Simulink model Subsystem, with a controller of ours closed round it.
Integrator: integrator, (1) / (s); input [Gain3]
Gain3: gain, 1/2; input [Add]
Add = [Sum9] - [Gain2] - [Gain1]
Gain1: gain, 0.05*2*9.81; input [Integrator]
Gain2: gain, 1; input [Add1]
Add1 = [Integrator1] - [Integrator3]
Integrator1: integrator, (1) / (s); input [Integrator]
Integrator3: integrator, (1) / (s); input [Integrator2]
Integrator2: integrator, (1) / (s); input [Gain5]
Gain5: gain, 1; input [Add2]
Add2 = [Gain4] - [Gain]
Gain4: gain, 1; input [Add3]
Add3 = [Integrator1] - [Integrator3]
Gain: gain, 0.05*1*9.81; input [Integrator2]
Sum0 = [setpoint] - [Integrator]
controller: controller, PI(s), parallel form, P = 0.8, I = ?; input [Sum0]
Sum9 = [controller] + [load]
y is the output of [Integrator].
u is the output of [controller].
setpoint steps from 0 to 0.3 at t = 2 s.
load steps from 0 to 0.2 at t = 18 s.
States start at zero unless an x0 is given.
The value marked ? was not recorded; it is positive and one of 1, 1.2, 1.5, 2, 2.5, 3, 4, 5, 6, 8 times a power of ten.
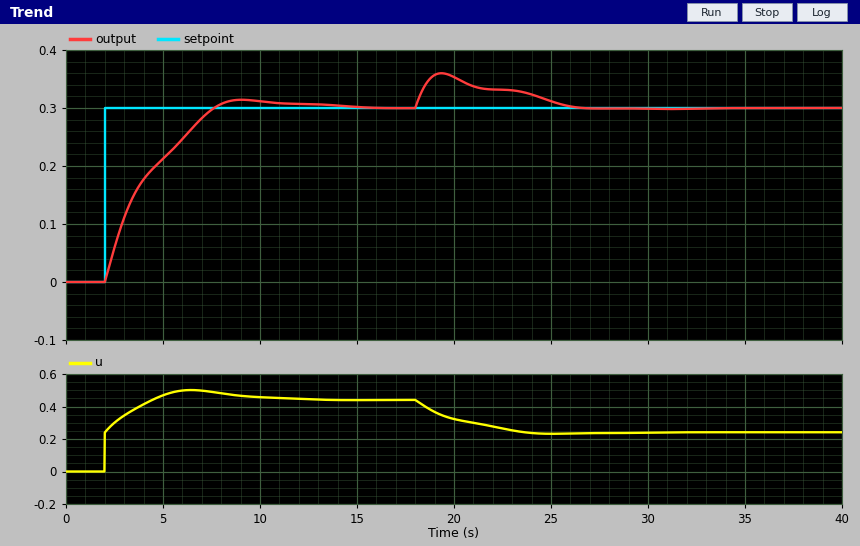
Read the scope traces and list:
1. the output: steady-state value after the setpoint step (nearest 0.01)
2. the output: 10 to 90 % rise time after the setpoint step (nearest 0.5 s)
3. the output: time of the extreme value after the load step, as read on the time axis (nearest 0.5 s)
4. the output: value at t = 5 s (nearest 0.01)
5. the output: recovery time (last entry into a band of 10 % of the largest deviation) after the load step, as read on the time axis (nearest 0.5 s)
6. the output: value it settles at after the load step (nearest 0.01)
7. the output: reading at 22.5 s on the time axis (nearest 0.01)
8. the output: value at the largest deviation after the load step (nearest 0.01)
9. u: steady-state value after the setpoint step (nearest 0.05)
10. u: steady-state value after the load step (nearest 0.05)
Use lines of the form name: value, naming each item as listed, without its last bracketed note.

the output: steady-state value after the setpoint step: 0.30
the output: 10 to 90 % rise time after the setpoint step: 4.5 s
the output: time of the extreme value after the load step, as read on the time axis: 19.5 s
the output: value at t = 5 s: 0.21
the output: recovery time (last entry into a band of 10 % of the largest deviation) after the load step, as read on the time axis: 25.5 s
the output: value it settles at after the load step: 0.30
the output: reading at 22.5 s on the time axis: 0.33
the output: value at the largest deviation after the load step: 0.36
u: steady-state value after the setpoint step: 0.45
u: steady-state value after the load step: 0.25
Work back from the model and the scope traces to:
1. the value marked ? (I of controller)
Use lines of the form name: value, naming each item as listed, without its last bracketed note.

the value marked ?: 0.8
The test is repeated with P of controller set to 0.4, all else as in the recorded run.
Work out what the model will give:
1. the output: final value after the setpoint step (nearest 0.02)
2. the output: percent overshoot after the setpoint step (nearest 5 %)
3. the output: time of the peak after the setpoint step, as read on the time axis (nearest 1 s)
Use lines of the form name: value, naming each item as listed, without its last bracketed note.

the output: final value after the setpoint step: 0.30
the output: percent overshoot after the setpoint step: 10 %
the output: time of the peak after the setpoint step, as read on the time axis: 9 s
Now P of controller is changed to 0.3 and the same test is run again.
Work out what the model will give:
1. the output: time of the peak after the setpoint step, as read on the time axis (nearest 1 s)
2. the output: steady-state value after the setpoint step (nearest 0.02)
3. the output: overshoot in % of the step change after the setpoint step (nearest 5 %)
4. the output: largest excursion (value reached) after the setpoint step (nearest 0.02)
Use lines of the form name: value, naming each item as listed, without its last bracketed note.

the output: time of the peak after the setpoint step, as read on the time axis: 9 s
the output: steady-state value after the setpoint step: 0.30
the output: overshoot in % of the step change after the setpoint step: 10 %
the output: largest excursion (value reached) after the setpoint step: 0.34
